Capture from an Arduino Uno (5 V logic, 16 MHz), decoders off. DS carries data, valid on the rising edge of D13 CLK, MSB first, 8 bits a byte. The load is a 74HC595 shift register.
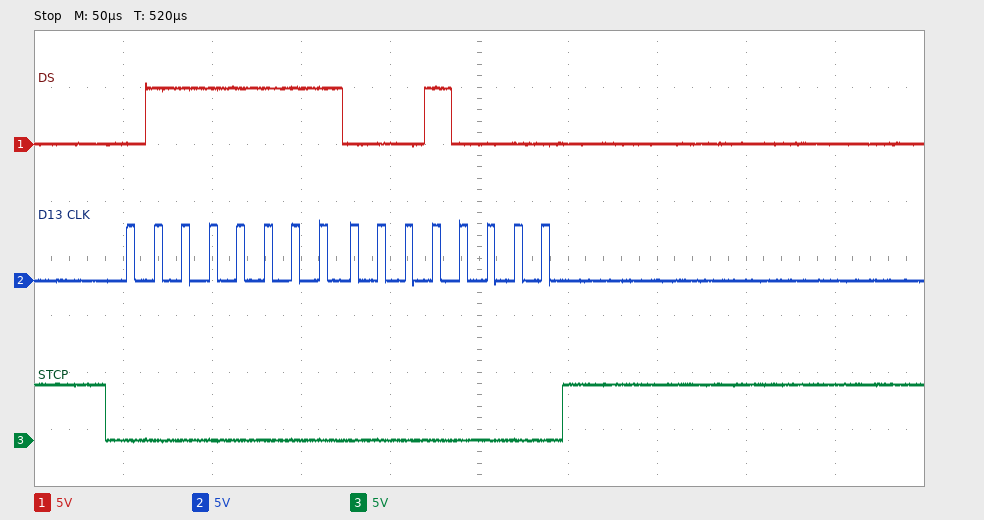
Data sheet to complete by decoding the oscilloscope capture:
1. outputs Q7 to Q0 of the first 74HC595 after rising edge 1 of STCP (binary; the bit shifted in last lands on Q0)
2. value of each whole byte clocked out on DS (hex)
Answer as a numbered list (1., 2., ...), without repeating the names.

1. 00010000
2. 7F 10
